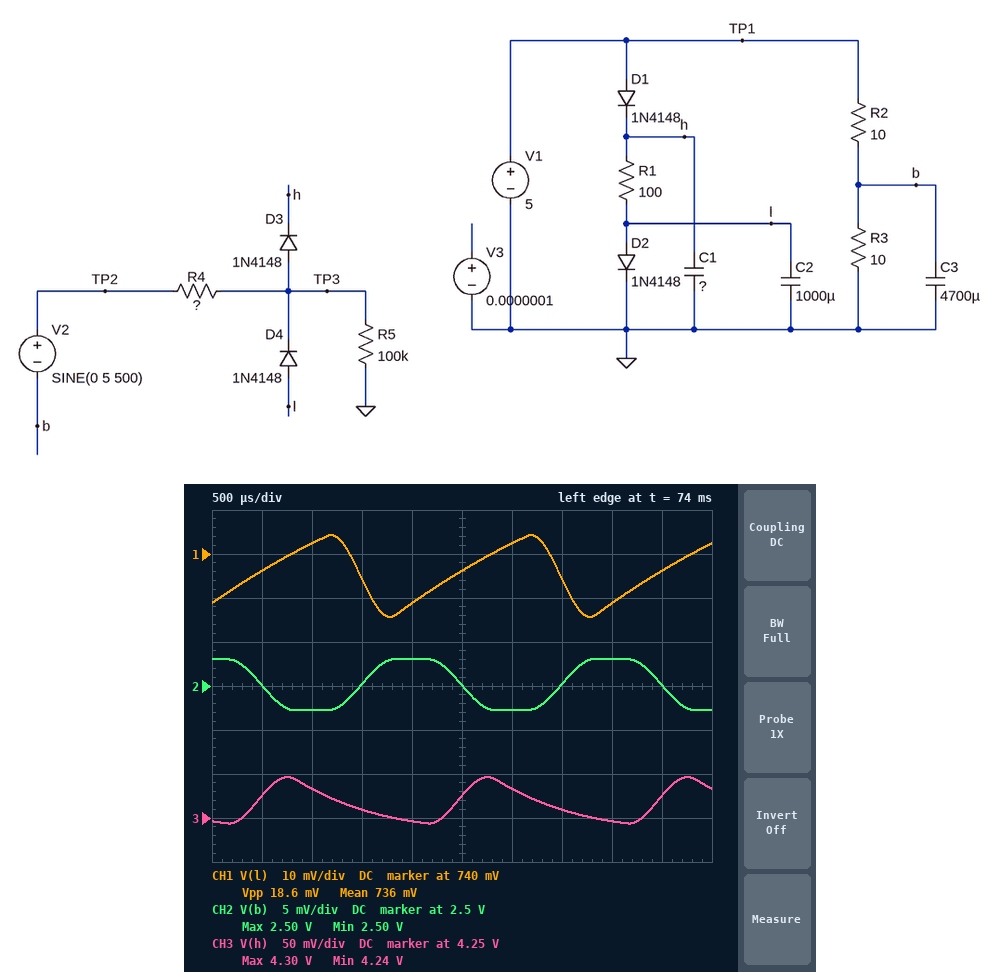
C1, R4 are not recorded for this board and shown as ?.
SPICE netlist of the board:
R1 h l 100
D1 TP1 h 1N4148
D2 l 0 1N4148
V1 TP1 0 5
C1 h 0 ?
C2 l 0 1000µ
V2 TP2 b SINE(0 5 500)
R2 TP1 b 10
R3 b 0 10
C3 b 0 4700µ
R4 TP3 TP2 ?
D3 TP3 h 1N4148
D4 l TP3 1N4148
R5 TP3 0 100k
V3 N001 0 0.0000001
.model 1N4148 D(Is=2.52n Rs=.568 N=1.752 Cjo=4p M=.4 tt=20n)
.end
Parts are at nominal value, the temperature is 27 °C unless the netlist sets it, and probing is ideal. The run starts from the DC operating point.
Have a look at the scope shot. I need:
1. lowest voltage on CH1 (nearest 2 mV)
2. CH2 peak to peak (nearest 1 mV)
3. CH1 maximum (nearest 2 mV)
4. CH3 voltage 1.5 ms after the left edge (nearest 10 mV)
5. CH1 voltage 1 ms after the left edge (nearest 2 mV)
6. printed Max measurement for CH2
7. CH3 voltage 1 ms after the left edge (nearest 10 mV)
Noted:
726 mV
6 mV
744 mV
4.26 V
742 mV
2.50 V
4.28 V
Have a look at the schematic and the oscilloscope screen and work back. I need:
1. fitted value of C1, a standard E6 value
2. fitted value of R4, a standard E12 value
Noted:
330 µF
39 Ω
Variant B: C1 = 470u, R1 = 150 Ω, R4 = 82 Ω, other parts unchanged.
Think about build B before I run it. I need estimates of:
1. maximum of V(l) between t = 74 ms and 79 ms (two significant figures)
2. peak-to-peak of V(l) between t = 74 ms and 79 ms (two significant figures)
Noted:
730 mV
9.0 mV
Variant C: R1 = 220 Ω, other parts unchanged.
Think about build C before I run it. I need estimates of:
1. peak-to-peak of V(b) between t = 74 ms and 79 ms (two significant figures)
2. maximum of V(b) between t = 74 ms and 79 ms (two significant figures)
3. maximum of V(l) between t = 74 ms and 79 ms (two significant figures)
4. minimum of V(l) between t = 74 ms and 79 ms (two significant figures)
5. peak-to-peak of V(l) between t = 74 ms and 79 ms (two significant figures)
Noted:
5.6 mV
2.5 V
660 mV
640 mV
18 mV
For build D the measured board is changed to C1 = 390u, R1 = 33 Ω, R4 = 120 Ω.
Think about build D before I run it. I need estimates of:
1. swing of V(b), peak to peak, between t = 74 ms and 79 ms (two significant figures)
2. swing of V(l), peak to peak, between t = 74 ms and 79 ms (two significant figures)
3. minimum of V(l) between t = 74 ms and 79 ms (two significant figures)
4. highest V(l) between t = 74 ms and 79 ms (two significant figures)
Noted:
2.1 mV
6.3 mV
840 mV
850 mV
